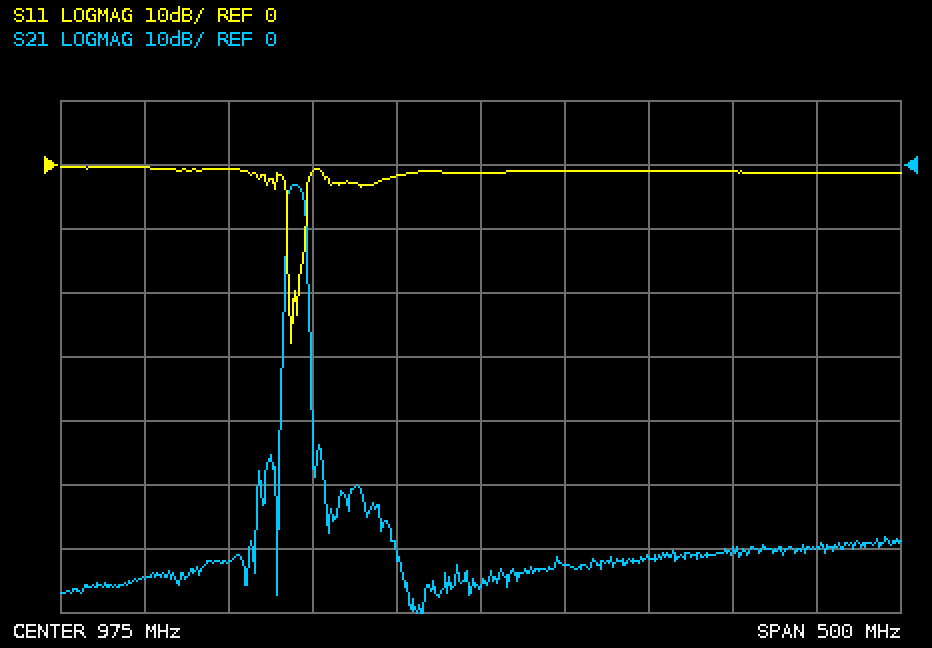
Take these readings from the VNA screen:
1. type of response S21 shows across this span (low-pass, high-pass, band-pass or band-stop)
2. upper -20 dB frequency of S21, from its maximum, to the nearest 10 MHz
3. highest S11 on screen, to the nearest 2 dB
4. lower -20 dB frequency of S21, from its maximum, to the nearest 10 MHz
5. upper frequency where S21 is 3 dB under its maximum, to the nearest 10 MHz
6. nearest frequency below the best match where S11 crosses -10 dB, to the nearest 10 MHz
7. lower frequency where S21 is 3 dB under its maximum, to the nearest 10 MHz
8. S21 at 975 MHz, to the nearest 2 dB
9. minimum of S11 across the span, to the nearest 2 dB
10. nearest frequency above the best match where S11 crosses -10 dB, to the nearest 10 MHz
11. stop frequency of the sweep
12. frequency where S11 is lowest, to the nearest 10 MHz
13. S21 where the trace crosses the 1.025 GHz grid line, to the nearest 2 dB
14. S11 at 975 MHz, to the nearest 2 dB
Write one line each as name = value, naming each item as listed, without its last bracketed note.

type of response S21 shows across this span = band-pass
upper -20 dB frequency of S21, from its maximum, to the nearest 10 MHz = 870 MHz
highest S11 on screen, to the nearest 2 dB = 0 dB
lower -20 dB frequency of S21, from its maximum, to the nearest 10 MHz = 860 MHz
upper frequency where S21 is 3 dB under its maximum, to the nearest 10 MHz = 870 MHz
nearest frequency below the best match where S11 crosses -10 dB, to the nearest 10 MHz = 860 MHz
lower frequency where S21 is 3 dB under its maximum, to the nearest 10 MHz = 860 MHz
S21 at 975 MHz, to the nearest 2 dB = -66 dB
minimum of S11 across the span, to the nearest 2 dB = -28 dB
nearest frequency above the best match where S11 crosses -10 dB, to the nearest 10 MHz = 870 MHz
stop frequency of the sweep = 1.225 GHz
frequency where S11 is lowest, to the nearest 10 MHz = 860 MHz
S21 where the trace crosses the 1.025 GHz grid line, to the nearest 2 dB = -62 dB
S11 at 975 MHz, to the nearest 2 dB = -2 dB
